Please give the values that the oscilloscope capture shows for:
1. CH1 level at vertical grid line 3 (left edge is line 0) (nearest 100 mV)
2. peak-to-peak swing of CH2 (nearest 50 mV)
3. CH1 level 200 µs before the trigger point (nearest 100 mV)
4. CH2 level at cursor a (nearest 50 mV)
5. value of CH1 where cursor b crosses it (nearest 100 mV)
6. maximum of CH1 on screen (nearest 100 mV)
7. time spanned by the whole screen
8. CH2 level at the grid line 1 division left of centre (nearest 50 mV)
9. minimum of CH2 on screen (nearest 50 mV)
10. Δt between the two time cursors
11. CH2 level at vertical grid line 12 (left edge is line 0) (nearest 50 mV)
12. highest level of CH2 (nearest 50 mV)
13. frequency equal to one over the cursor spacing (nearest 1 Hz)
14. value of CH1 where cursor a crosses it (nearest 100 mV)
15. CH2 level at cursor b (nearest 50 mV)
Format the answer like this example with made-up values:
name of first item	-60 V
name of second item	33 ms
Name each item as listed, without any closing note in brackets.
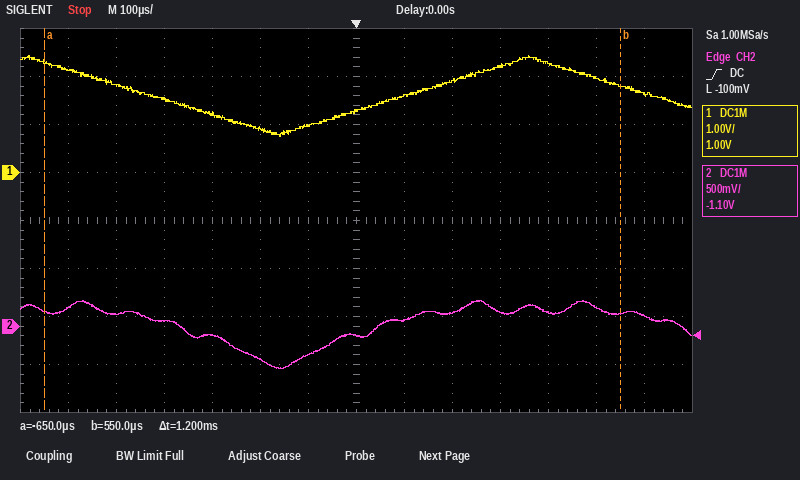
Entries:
CH1 level at vertical grid line 3 (left edge is line 0)	1.5 V
peak-to-peak swing of CH2	700 mV
CH1 level 200 µs before the trigger point	900 mV
CH2 level at cursor a	150 mV
value of CH1 where cursor b crosses it	1.8 V
maximum of CH1 on screen	2.4 V
time spanned by the whole screen	1.4 ms
CH2 level at the grid line 1 division left of centre	-300 mV
minimum of CH2 on screen	-450 mV
Δt between the two time cursors	1.2 ms
CH2 level at vertical grid line 12 (left edge is line 0)	200 mV
highest level of CH2	250 mV
frequency equal to one over the cursor spacing	833 Hz
value of CH1 where cursor a crosses it	2.3 V
CH2 level at cursor b	150 mV
